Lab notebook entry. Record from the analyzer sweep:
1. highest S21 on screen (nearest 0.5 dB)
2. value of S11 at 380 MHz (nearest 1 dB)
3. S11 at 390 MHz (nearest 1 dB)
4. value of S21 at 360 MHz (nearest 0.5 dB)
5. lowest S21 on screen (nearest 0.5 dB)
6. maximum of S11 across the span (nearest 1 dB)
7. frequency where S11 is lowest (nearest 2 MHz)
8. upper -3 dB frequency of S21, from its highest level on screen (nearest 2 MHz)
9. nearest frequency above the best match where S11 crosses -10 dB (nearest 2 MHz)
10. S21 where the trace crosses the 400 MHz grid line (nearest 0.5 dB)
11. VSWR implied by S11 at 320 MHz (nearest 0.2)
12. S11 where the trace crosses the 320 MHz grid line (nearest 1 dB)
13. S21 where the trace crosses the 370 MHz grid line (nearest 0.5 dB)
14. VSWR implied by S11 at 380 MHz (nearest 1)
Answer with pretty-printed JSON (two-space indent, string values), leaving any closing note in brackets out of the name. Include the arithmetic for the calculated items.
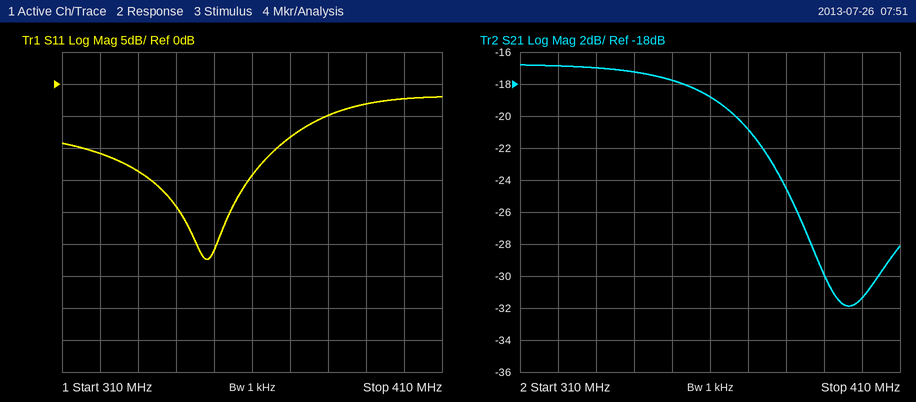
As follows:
{
  "highest S21 on screen": "-17.0 dB",
  "value of S11 at 380 MHz": "-5 dB",
  "S11 at 390 MHz": "-3 dB",
  "value of S21 at 360 MHz": "-19.0 dB",
  "lowest S21 on screen": "-32.0 dB",
  "maximum of S11 across the span": "-2 dB",
  "frequency where S11 is lowest": "348 MHz",
  "upper -3 dB frequency of S21, from its highest level on screen": "366 MHz",
  "nearest frequency above the best match where S11 crosses -10 dB": "366 MHz",
  "S21 where the trace crosses the 400 MHz grid line": "-31.5 dB",
  "VSWR implied by S11 at 320 MHz": "|Γ| = 10^(-11/20) = 0.2818; VSWR = (1 + 0.2818)/(1 − 0.2818) ≈ 1.8",
  "S11 where the trace crosses the 320 MHz grid line": "-11 dB",
  "S21 where the trace crosses the 370 MHz grid line": "-21.0 dB",
  "VSWR implied by S11 at 380 MHz": "|Γ| = 10^(-5/20) = 0.5623; VSWR = (1 + 0.5623)/(1 − 0.5623) ≈ 4"
}
